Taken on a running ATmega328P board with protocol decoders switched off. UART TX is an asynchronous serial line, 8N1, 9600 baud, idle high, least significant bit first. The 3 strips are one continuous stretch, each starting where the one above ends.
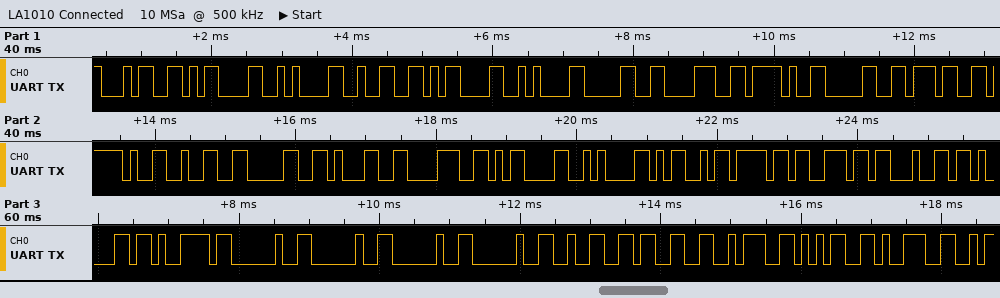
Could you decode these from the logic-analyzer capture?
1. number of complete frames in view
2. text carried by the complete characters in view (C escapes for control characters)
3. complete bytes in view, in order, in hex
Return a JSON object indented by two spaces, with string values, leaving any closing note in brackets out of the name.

{
  "number of complete frames in view": "33",
  "text carried by the complete characters in view": "\"4\\r\\n2\\r\\n08/07/2018\\r\\nMonday    23:59\"",
  "complete bytes in view, in order, in hex": "0x34 0x0D 0x0A 0x32 0x0D 0x0A 0x30 0x38 0x2F 0x30 0x37 0x2F 0x32 0x30 0x31 0x38 0x0D 0x0A 0x4D 0x6F 0x6E 0x64 0x61 0x79 0x20 0x20 0x20 0x20 0x32 0x33 0x3A 0x35 0x39"
}
